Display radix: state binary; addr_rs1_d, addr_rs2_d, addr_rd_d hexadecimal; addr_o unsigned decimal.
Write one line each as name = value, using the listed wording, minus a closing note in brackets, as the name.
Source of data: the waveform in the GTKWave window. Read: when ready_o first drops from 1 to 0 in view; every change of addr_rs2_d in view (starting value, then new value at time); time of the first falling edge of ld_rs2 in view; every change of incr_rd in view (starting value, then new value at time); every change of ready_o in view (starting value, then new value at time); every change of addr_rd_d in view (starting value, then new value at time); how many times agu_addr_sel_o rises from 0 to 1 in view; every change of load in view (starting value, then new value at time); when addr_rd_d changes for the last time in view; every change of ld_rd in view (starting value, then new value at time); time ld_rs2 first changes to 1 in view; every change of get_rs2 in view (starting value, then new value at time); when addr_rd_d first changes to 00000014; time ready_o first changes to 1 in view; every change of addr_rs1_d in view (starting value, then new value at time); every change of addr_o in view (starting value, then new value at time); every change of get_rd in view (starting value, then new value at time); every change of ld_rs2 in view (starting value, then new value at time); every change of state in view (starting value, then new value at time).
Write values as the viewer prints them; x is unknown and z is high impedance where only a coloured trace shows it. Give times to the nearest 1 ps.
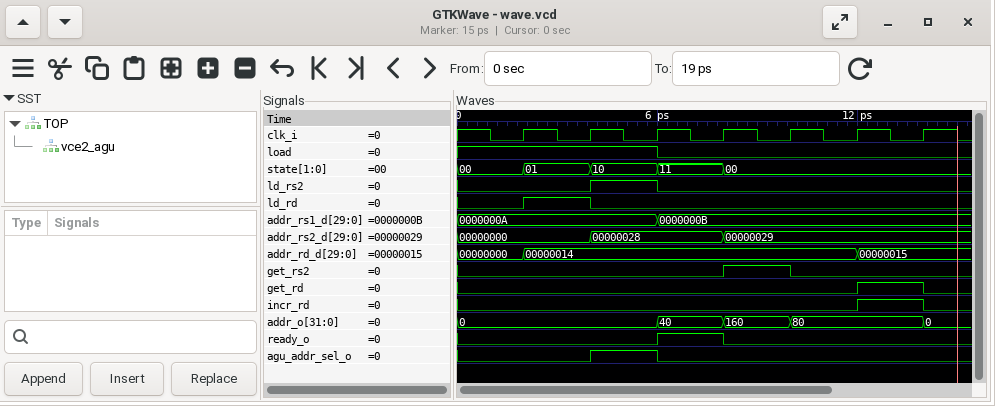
when ready_o first drops from 1 to 0 in view = 8 ps
every change of addr_rs2_d in view = 00000000, 00000028 at 4 ps, 00000029 at 8 ps
time of the first falling edge of ld_rs2 in view = 6 ps
every change of incr_rd in view = 0, 1 at 12 ps, 0 at 14 ps
every change of ready_o in view = 0, 1 at 6 ps, 0 at 8 ps
every change of addr_rd_d in view = 00000000, 00000014 at 2 ps, 00000015 at 12 ps
how many times agu_addr_sel_o rises from 0 to 1 in view = 1
every change of load in view = 1, 0 at 6 ps
when addr_rd_d changes for the last time in view = 12 ps
every change of ld_rd in view = 0, 1 at 2 ps, 0 at 4 ps
time ld_rs2 first changes to 1 in view = 4 ps
every change of get_rs2 in view = 0, 1 at 8 ps, 0 at 10 ps
when addr_rd_d first changes to 00000014 = 2 ps
time ready_o first changes to 1 in view = 6 ps
every change of addr_rs1_d in view = 0000000A, 0000000B at 6 ps
every change of addr_o in view = 0, 40 at 6 ps, 160 at 8 ps, 80 at 10 ps, 0 at 14 ps
every change of get_rd in view = 0, 1 at 12 ps, 0 at 14 ps
every change of ld_rs2 in view = 0, 1 at 4 ps, 0 at 6 ps
every change of state in view = 00, 01 at 2 ps, 10 at 4 ps, 11 at 6 ps, 00 at 8 ps
